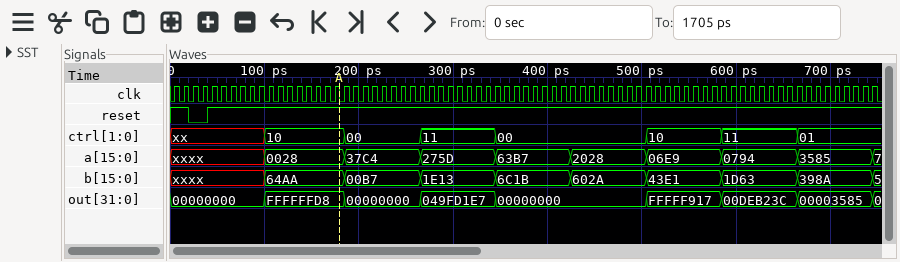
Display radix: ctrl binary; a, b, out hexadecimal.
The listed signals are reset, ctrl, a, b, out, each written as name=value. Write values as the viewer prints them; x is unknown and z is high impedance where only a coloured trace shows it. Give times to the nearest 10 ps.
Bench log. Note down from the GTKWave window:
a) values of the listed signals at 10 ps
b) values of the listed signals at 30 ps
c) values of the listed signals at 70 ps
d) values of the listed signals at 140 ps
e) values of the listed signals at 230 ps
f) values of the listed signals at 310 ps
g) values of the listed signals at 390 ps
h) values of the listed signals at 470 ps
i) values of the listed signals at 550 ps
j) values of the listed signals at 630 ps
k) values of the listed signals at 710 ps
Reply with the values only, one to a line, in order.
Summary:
reset=1, ctrl=xx, a=xxxx, b=xxxx, out=00000000
reset=0, ctrl=xx, a=xxxx, b=xxxx, out=00000000
reset=1, ctrl=xx, a=xxxx, b=xxxx, out=00000000
reset=1, ctrl=10, a=0028, b=64AA, out=FFFFFFD8
reset=1, ctrl=00, a=37C4, b=00B7, out=00000000
reset=1, ctrl=11, a=275D, b=1E13, out=049FD1E7
reset=1, ctrl=00, a=63B7, b=6C1B, out=00000000
reset=1, ctrl=00, a=2028, b=602A, out=00000000
reset=1, ctrl=10, a=06E9, b=43E1, out=FFFFF917
reset=1, ctrl=11, a=0794, b=1D63, out=00DEB23C
reset=1, ctrl=01, a=3585, b=398A, out=00003585
